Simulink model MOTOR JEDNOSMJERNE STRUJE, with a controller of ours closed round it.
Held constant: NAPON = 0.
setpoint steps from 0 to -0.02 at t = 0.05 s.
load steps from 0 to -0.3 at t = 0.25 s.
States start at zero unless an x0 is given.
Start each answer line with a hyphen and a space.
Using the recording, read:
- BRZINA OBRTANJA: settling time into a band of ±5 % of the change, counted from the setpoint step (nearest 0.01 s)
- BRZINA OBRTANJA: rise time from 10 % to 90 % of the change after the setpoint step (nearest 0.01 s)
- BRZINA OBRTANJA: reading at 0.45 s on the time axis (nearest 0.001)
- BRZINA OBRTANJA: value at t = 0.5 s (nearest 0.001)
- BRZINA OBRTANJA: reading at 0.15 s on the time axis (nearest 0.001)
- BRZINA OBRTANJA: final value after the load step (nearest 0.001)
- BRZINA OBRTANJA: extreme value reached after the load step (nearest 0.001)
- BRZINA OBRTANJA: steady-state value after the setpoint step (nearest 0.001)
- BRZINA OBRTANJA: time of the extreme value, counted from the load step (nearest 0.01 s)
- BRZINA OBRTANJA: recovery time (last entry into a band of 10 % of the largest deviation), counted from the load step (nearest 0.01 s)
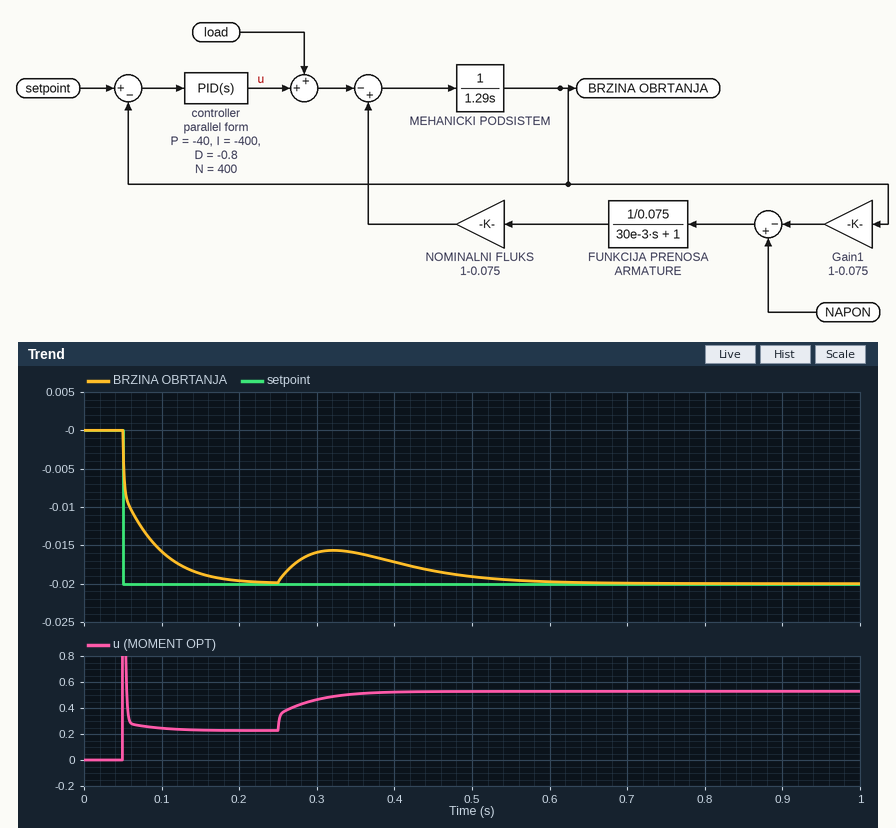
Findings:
- 0.11 s
- 0.08 s
- -0.018
- -0.019
- -0.019
- -0.020
- -0.016
- -0.020
- 0.07 s
- 0.31 s
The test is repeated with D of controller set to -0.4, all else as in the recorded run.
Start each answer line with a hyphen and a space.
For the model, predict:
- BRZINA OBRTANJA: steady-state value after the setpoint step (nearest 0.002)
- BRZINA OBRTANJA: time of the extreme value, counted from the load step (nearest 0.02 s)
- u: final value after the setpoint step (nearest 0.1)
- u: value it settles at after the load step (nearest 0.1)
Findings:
- -0.020
- 0.06 s
- 0.2
- 0.5
